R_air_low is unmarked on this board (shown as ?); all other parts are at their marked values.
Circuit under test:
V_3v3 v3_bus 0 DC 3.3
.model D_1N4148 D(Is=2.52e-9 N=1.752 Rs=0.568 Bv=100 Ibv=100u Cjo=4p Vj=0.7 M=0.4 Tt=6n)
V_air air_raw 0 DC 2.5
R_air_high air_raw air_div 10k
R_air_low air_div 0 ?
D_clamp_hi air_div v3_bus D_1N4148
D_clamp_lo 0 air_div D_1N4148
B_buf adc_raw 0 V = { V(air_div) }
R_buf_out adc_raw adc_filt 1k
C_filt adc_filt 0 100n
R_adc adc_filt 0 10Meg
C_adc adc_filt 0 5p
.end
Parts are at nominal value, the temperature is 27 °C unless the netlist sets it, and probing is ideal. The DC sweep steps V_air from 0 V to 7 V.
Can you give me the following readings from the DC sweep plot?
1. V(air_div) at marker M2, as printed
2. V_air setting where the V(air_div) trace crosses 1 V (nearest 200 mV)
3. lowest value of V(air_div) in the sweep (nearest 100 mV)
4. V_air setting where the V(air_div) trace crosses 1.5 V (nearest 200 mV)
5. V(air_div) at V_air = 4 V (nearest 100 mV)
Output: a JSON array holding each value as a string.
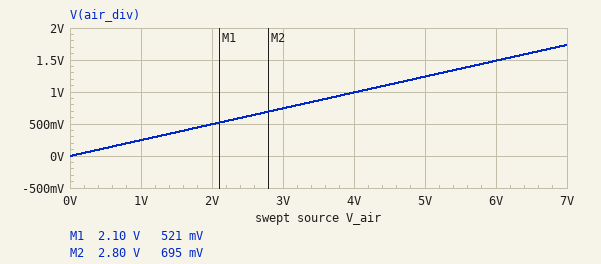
["695 mV", "4.0 V", "0 V", "6.0 V", "1.0 V"]
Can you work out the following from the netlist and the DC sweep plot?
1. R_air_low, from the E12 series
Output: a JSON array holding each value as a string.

["3.3 kΩ"]
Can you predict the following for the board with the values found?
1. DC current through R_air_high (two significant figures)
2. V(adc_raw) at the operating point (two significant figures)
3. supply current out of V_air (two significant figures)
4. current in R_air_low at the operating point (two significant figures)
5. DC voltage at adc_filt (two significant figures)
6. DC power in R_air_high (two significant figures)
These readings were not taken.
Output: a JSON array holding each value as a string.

["190 µA", "620 mV", "190 µA", "190 µA", "620 mV", "350 µW"]
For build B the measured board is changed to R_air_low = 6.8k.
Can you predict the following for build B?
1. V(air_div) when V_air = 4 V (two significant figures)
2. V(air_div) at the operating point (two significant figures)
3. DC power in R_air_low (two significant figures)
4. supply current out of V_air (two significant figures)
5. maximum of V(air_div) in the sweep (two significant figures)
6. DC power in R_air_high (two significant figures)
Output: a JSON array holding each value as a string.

["1.6 V", "1.0 V", "150 µW", "150 µA", "2.8 V", "220 µW"]
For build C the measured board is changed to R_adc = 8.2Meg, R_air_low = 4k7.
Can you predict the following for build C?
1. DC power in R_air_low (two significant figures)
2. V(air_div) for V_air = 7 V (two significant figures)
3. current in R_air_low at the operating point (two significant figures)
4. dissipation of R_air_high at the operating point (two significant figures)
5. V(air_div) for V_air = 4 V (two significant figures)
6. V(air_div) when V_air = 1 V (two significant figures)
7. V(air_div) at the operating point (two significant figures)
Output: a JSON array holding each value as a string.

["140 µW", "2.2 V", "170 µA", "290 µW", "1.3 V", "320 mV", "800 mV"]
